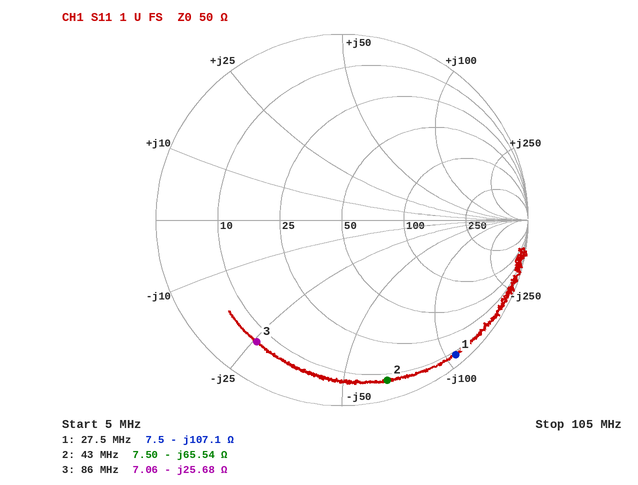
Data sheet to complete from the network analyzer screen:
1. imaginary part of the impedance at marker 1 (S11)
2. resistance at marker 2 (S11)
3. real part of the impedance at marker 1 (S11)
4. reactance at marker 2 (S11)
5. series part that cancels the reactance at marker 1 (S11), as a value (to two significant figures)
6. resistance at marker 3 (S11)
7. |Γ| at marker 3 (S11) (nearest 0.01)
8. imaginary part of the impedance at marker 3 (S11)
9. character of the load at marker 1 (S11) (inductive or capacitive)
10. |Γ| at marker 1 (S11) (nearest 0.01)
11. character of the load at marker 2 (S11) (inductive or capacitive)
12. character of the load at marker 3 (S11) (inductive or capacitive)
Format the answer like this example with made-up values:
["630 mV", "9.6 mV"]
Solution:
["-107.1 Ω", "7.50 Ω", "7.5 Ω", "-65.54 Ω", "620 nH", "7.06 Ω", "0.80", "-25.68 Ω", "capacitive", "0.95", "capacitive", "capacitive"]
